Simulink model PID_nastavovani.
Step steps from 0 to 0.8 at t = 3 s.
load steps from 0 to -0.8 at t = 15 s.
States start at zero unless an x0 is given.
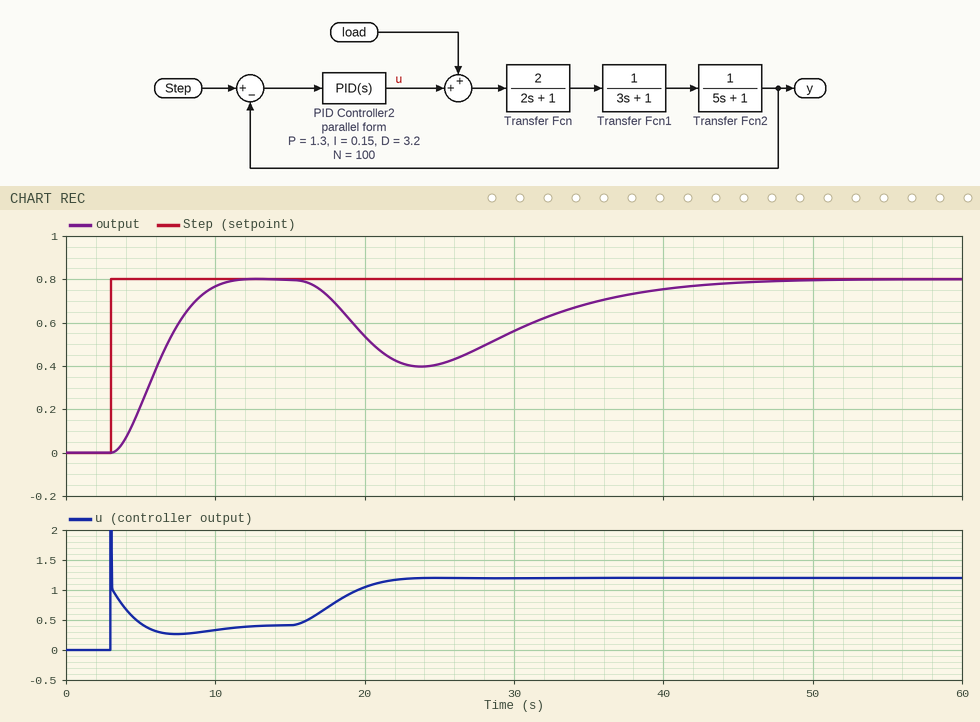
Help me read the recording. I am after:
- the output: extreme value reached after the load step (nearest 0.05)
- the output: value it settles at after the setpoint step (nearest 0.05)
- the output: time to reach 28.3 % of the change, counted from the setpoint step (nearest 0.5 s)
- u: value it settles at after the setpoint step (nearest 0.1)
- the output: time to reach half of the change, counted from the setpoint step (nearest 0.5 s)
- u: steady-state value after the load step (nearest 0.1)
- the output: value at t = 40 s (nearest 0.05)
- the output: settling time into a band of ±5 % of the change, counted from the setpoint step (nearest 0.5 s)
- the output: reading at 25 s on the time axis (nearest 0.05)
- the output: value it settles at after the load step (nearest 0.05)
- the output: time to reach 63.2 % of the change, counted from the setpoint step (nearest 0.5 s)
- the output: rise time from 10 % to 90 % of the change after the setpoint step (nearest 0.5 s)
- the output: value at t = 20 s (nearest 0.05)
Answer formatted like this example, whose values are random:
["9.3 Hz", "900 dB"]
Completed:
["0.40", "0.80", "2.0 s", "0.4", "3.0 s", "1.2", "0.75", "7.0 s", "0.40", "0.80", "4.0 s", "5.0 s", "0.55"]
